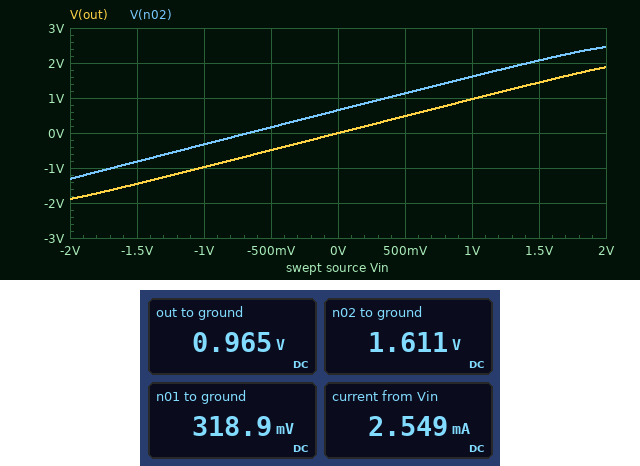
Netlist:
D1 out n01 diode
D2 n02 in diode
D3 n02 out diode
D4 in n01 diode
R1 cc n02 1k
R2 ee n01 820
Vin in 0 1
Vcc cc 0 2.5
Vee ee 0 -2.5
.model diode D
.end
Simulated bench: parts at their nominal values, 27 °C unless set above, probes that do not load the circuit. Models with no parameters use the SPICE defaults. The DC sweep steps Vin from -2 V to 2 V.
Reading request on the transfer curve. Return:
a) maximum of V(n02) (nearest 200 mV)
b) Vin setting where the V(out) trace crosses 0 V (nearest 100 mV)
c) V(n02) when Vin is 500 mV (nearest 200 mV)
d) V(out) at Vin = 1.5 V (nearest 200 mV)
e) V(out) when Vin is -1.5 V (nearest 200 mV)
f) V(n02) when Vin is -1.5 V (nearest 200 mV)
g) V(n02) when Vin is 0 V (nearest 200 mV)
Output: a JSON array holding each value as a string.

["2.4 V", "0 V", "1.2 V", "1.4 V", "-1.4 V", "-800 mV", "600 mV"]
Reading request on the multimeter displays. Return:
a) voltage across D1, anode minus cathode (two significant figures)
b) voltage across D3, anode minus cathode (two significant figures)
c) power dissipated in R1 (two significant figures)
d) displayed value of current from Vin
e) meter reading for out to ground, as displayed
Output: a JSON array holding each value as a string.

["650 mV", "650 mV", "790 µW", "2.549 mA", "0.965 V"]
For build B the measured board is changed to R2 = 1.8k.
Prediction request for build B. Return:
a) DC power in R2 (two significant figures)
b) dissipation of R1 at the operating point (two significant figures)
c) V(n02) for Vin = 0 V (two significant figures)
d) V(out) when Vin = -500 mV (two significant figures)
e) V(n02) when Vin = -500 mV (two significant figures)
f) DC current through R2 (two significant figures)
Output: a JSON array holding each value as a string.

["4.5 mW", "770 µW", "660 mV", "-470 mV", "170 mV", "1.6 mA"]
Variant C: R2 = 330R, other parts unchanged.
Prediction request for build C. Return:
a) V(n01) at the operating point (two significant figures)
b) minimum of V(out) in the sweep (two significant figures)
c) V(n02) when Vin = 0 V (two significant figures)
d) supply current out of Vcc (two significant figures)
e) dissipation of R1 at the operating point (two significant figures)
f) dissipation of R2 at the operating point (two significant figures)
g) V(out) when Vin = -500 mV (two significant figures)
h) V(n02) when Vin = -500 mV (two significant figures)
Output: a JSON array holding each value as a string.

["290 mV", "-1.9 V", "640 mV", "910 µA", "820 µW", "24 mW", "-510 mV", "150 mV"]
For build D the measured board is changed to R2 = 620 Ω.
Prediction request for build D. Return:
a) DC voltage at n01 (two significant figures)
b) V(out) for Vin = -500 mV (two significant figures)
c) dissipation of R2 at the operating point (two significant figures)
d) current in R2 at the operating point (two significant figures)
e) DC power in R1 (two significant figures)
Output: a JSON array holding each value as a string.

["310 mV", "-500 mV", "13 mW", "4.5 mA", "800 µW"]
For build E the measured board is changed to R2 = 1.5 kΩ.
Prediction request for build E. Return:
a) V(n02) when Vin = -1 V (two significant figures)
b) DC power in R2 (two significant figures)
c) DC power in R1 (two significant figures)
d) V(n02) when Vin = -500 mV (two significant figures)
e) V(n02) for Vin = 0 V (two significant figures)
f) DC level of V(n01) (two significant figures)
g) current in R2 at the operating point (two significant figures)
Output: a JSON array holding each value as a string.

["-320 mV", "5.4 mW", "770 µW", "170 mV", "660 mV", "340 mV", "1.9 mA"]
